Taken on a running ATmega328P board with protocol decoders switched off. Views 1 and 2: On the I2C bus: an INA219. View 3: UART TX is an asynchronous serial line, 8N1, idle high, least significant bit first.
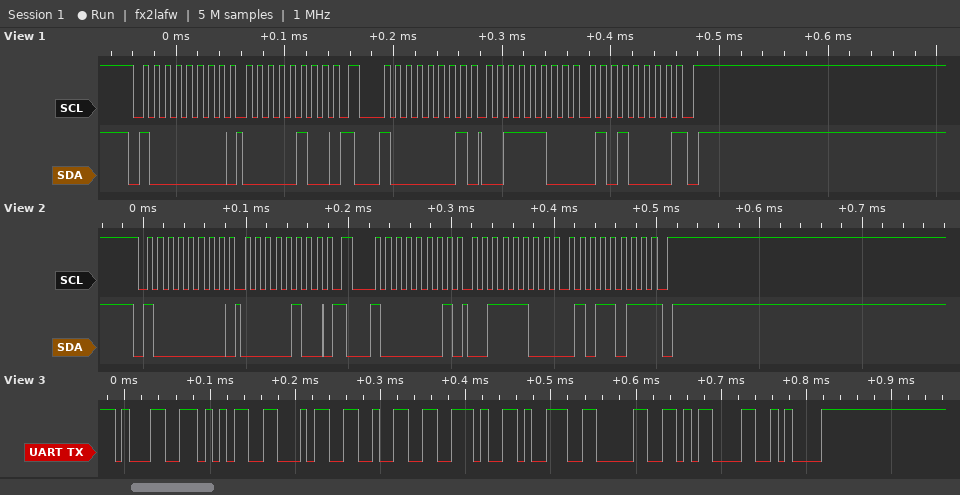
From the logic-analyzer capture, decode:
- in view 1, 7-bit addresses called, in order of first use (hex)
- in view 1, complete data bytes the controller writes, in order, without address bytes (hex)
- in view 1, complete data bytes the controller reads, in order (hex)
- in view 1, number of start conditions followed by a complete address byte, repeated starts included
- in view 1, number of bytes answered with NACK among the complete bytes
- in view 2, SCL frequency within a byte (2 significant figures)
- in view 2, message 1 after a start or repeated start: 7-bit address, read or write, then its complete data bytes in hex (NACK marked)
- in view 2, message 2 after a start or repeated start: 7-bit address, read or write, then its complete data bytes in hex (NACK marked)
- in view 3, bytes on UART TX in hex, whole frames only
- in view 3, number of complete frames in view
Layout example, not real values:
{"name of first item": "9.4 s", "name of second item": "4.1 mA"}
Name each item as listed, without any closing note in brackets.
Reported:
{"in view 1, 7-bit addresses called, in order of first use": "0x40", "in view 1, complete data bytes the controller writes, in order, without address bytes": "04", "in view 1, complete data bytes the controller reads, in order": "3C 50", "in view 1, number of start conditions followed by a complete address byte, repeated starts included": "2", "in view 1, number of bytes answered with NACK among the complete bytes": "1", "in view 2, SCL frequency within a byte": "100 kHz", "in view 2, message 1 after a start or repeated start: 7-bit address, read or write, then its complete data bytes in hex": "0x40 write: 04", "in view 2, message 2 after a start or repeated start: 7-bit address, read or write, then its complete data bytes in hex": "0x40 read: 3C 5B NACK", "in view 3, bytes on UART TX in hex, whole frames only": "31 35 34 32 2E 39 30 0D 0A", "in view 3, number of complete frames in view": "9"}
